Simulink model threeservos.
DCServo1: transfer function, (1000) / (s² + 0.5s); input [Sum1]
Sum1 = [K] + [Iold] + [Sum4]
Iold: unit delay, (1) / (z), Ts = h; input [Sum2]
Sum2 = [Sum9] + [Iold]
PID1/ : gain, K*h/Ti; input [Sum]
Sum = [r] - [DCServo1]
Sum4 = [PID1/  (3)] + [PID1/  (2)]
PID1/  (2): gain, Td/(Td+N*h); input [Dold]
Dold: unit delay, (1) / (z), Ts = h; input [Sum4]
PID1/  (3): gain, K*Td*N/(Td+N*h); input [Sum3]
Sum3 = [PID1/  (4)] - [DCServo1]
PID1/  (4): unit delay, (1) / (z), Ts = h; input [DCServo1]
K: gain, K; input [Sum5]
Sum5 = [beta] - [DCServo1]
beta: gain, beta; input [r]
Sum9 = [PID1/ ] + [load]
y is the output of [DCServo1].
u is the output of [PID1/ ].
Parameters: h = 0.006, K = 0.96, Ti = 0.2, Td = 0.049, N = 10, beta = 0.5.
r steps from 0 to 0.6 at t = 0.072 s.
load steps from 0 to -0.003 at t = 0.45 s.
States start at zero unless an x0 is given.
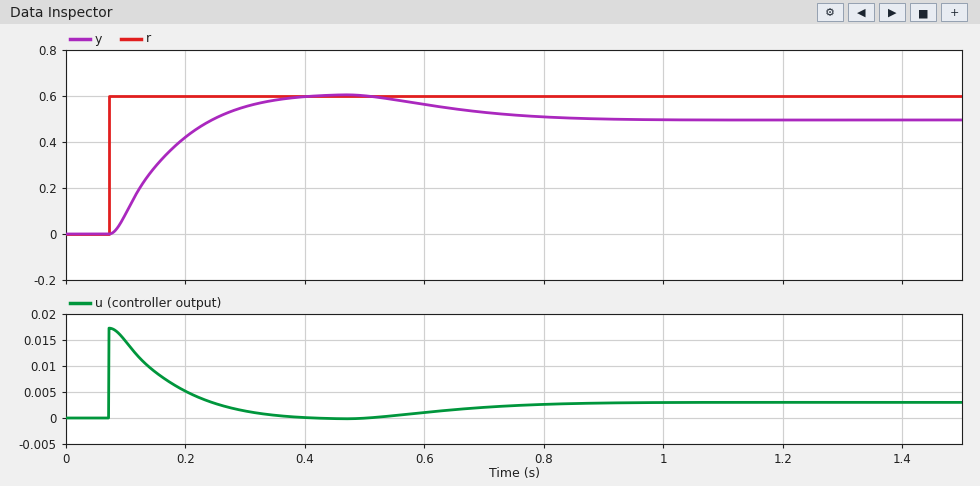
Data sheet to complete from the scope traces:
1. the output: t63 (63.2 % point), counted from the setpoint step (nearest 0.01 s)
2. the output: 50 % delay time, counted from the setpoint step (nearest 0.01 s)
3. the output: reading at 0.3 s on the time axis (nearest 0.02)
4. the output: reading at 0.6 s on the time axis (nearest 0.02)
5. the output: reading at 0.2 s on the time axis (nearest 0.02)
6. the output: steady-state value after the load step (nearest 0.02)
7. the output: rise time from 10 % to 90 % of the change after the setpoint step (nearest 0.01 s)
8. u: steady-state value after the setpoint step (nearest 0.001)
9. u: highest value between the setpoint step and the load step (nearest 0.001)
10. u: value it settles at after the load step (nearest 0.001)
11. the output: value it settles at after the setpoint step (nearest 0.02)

0.11 s
0.08 s
0.56
0.56
0.42
0.50
0.19 s
0.000
0.017
0.003
0.60
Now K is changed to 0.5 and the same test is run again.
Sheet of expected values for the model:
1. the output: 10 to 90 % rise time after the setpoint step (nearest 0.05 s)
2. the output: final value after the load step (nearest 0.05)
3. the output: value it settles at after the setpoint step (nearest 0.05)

0.15 s
0.40
0.60
